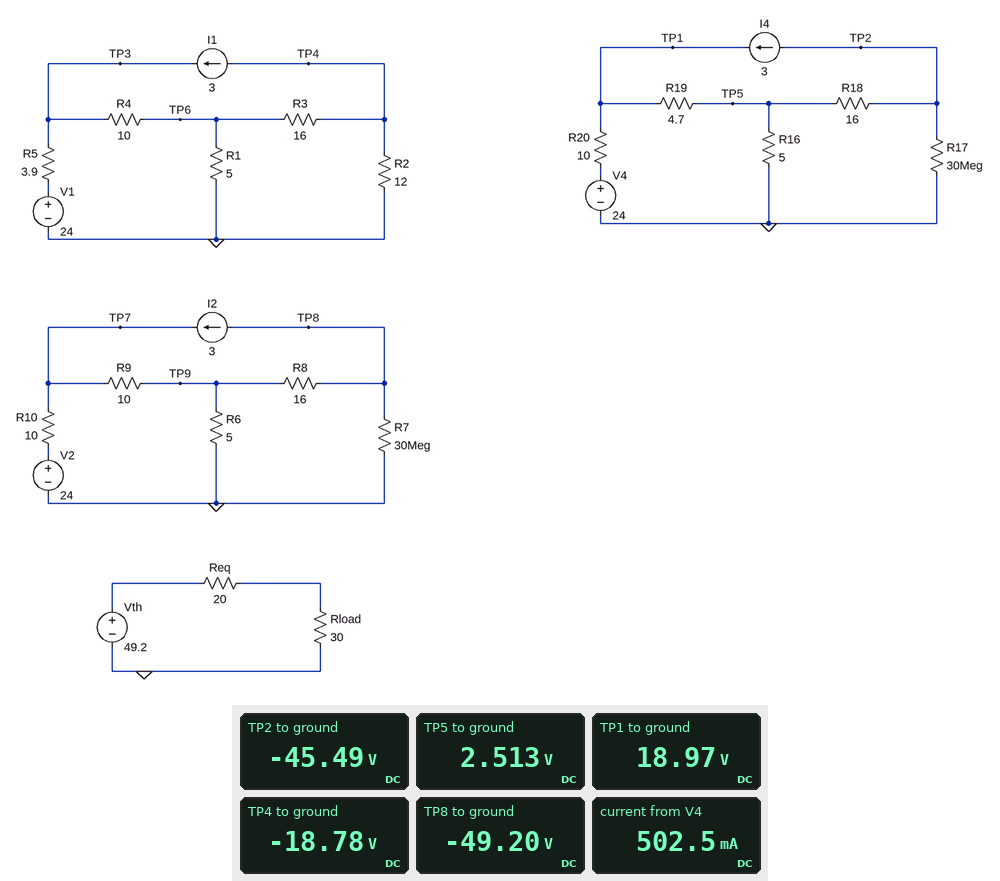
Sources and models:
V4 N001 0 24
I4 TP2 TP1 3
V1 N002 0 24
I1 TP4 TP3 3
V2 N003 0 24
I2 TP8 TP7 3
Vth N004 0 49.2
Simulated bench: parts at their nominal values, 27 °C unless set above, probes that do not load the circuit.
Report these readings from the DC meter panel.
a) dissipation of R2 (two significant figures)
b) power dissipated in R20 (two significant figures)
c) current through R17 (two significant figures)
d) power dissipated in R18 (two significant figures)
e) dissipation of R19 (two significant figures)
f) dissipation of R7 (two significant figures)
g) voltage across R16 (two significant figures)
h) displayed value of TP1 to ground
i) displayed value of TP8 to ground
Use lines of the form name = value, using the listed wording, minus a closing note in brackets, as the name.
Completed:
dissipation of R2 = 29 W
power dissipated in R20 = 2.5 W
current through R17 = 1.5 µA
power dissipated in R18 = 140 W
dissipation of R19 = 58 W
dissipation of R7 = 81 µW
voltage across R16 = 2.5 V
displayed value of TP1 to ground = 18.97 V
displayed value of TP8 to ground = -49.20 V
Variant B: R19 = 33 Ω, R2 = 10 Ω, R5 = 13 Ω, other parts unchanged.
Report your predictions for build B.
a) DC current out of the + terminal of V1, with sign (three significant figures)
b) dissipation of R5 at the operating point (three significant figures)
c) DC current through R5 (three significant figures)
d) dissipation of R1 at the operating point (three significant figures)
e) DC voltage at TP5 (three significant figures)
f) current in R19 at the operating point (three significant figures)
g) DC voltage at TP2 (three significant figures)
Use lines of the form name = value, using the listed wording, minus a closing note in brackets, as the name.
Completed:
DC current out of the + terminal of V1, with sign = -505 mA
dissipation of R5 at the operating point = 3.32 W
DC current through R5 = 505 mA
dissipation of R1 at the operating point = 6.32 W
DC voltage at TP5 = -7.81 V
current in R19 at the operating point = 1.44 A
DC voltage at TP2 = -55.8 V
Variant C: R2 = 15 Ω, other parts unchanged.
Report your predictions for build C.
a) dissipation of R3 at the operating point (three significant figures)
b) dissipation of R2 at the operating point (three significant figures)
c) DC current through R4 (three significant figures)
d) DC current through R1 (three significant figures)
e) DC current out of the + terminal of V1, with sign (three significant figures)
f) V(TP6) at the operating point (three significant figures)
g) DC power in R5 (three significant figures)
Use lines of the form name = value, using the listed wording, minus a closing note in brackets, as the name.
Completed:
dissipation of R3 at the operating point = 39.4 W
dissipation of R2 at the operating point = 30.7 W
DC current through R4 = 2.30 A
DC current through R1 = 734 mA
DC current out of the + terminal of V1, with sign = -696 mA
V(TP6) at the operating point = 3.67 V
DC power in R5 = 1.89 W
